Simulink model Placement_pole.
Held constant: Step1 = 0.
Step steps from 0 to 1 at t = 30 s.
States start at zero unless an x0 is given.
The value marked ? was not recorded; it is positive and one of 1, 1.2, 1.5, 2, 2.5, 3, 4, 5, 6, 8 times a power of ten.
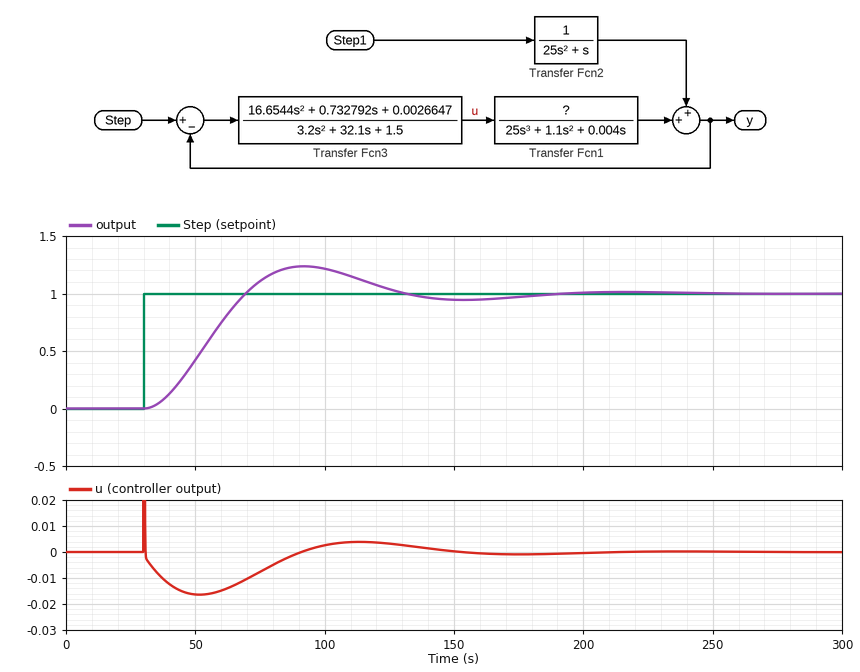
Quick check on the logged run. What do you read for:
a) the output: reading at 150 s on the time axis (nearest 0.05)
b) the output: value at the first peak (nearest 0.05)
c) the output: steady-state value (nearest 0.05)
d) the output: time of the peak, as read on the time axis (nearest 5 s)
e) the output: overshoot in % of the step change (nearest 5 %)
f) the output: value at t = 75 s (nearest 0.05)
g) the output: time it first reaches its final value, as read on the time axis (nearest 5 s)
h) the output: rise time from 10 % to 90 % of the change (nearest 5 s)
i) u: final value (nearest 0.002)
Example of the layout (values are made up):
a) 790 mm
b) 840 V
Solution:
a) 0.95
b) 1.25
c) 1.00
d) 90 s
e) 25 %
f) 1.10
g) 70 s
h) 25 s
i) 0.000
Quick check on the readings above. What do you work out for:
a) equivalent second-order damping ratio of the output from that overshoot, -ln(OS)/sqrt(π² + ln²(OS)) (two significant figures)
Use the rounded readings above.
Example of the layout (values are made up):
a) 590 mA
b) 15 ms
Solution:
a) 0.40
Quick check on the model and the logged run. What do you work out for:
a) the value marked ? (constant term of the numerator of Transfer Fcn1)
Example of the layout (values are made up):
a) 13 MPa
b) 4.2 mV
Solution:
a) 0.15
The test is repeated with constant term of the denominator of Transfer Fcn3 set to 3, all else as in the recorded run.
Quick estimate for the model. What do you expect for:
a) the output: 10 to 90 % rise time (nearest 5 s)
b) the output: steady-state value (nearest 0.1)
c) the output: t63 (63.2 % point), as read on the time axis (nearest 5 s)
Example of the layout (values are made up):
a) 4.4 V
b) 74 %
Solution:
a) 45 s
b) 1.0
c) 65 s
